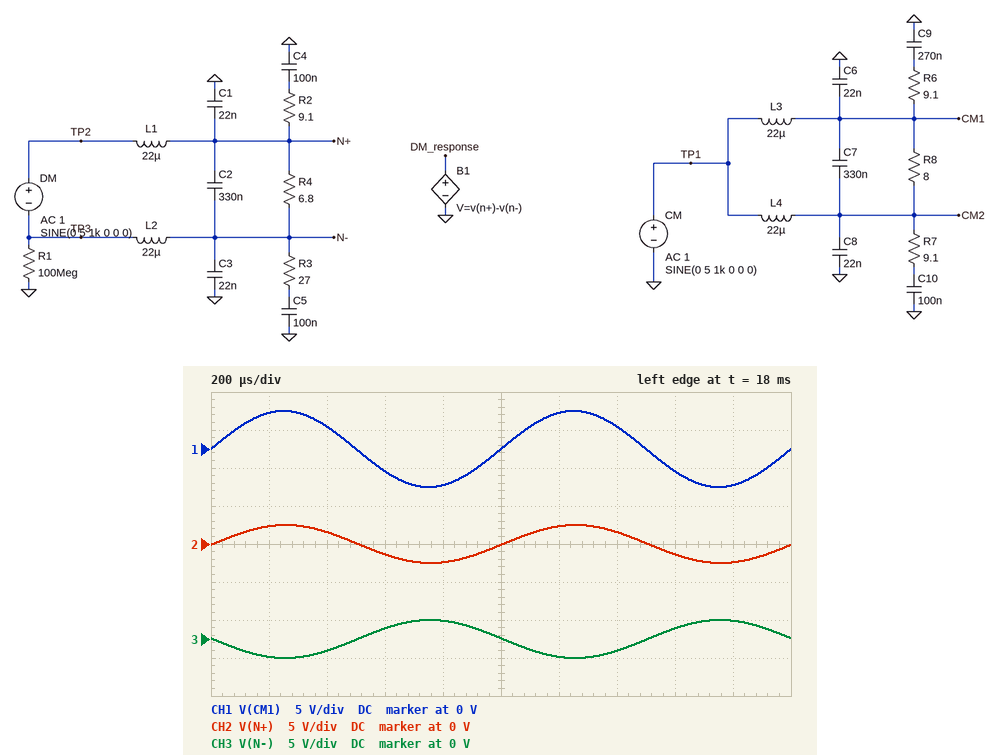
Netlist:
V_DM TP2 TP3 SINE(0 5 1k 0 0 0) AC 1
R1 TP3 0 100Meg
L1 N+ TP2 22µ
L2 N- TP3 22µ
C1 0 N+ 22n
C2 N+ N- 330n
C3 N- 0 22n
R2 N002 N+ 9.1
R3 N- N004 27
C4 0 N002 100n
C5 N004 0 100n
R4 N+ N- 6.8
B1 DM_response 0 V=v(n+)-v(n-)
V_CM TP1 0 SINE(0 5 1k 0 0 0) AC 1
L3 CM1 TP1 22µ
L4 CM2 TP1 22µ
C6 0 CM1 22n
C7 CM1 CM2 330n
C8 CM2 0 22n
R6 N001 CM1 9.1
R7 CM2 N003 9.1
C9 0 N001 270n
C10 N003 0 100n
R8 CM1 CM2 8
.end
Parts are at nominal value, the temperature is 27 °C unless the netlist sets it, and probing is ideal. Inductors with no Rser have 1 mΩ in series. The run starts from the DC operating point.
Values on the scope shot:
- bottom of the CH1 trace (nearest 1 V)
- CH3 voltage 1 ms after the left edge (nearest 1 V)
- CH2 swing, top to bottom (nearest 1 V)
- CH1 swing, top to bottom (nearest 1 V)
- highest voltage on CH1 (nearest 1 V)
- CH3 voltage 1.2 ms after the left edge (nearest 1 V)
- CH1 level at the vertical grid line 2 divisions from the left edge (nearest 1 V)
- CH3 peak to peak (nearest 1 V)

-5 V
0 V
5 V
10 V
5 V
-2 V
3 V
5 V
